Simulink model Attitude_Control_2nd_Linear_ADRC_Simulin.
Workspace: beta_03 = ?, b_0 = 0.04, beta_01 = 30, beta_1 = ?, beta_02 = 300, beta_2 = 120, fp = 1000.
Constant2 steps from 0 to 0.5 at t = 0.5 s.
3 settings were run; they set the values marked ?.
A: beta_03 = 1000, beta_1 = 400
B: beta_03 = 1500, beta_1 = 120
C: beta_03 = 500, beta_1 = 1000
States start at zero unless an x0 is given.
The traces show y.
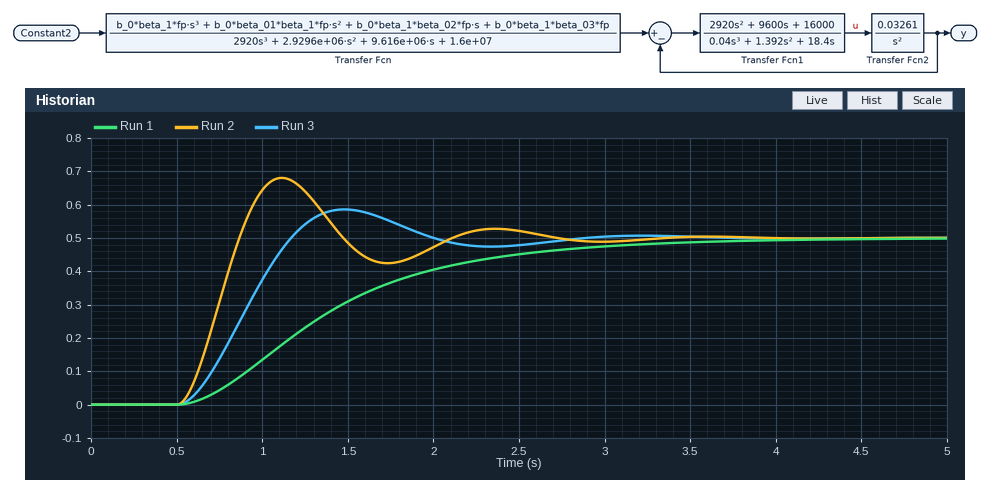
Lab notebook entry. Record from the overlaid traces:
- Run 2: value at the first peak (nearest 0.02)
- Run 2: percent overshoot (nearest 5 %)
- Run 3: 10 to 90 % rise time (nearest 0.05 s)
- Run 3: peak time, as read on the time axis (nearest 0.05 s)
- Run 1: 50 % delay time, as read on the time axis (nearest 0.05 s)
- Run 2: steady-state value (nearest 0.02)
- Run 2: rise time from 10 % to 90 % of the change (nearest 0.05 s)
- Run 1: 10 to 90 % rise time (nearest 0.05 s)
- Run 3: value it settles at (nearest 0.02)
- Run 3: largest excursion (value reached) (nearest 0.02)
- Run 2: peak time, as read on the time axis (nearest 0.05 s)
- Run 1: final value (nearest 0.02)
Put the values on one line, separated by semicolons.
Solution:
0.68; 35 %; 0.45 s; 1.50 s; 1.30 s; 0.50; 0.25 s; 1.70 s; 0.50; 0.58; 1.10 s; 0.50
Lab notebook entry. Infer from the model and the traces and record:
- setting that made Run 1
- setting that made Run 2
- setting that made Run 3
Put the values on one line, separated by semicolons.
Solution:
B; C; A
